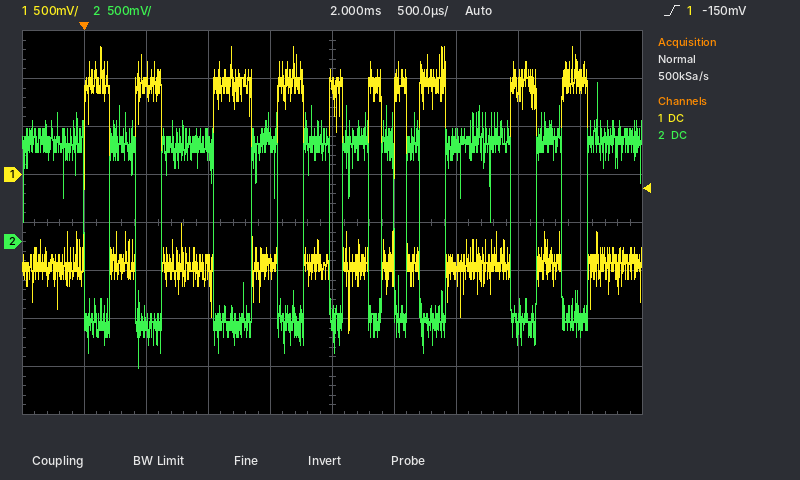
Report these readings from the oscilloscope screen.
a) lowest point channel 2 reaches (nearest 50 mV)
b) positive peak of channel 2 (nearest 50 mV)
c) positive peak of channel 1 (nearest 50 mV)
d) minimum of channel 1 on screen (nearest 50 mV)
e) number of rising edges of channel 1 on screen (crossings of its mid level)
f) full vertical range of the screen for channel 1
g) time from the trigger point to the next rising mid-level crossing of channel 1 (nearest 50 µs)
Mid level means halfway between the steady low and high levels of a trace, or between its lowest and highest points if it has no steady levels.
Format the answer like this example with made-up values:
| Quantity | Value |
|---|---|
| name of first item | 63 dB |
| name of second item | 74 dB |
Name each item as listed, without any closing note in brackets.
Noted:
| Quantity | Value |
|---|---|
| lowest point channel 2 reaches | -1.30 V |
| positive peak of channel 2 | 1.65 V |
| positive peak of channel 1 | 1.35 V |
| minimum of channel 1 on screen | -1.65 V |
| number of rising edges of channel 1 on screen | 10 |
| full vertical range of the screen for channel 1 | 4 V |
| time from the trigger point to the next rising mid-level crossing of channel 1 | 400 µs |
